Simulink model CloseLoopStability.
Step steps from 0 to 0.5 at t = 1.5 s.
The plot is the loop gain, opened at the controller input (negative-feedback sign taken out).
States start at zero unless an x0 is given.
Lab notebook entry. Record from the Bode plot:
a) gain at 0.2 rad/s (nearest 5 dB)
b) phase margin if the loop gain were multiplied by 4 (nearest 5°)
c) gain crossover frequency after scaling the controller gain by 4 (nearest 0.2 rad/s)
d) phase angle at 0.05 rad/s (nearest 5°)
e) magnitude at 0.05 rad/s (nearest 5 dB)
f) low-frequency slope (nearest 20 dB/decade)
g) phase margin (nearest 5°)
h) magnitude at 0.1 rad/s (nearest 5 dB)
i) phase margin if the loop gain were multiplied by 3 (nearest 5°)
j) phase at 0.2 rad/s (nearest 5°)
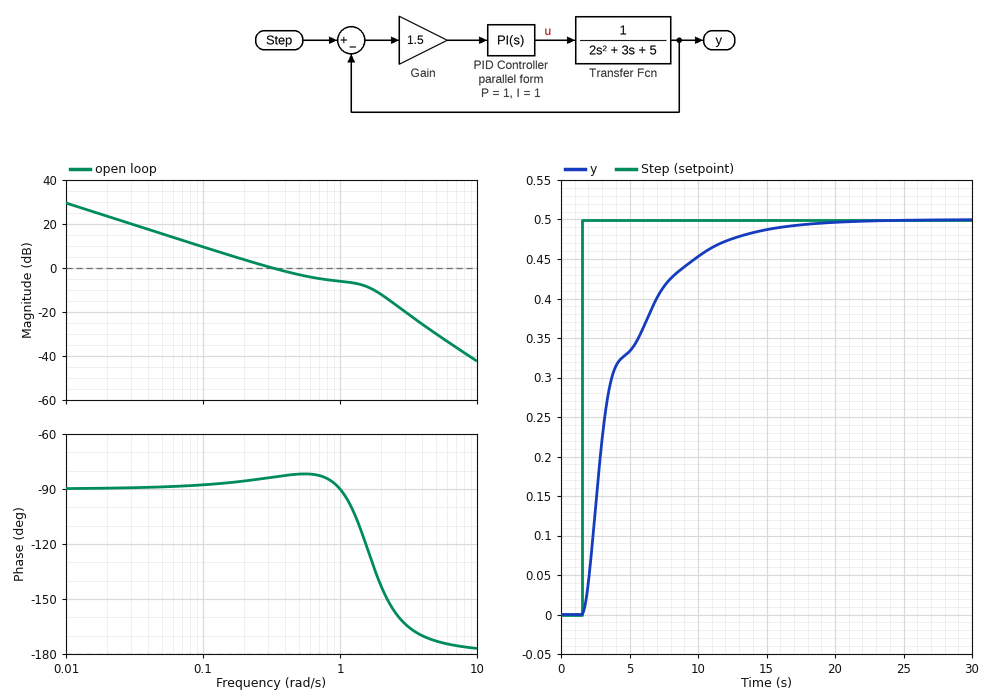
5 dB
35°
2.0 rad/s
-90°
15 dB
-20 dB/decade
95°
10 dB
50°
-85°
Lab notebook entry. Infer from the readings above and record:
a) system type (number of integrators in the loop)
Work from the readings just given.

1
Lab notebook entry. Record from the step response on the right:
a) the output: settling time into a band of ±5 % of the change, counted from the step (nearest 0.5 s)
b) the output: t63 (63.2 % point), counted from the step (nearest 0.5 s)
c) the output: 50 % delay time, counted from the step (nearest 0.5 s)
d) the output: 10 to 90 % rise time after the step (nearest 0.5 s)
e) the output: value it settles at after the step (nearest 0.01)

11.0 s
2.5 s
1.5 s
7.5 s
0.50
